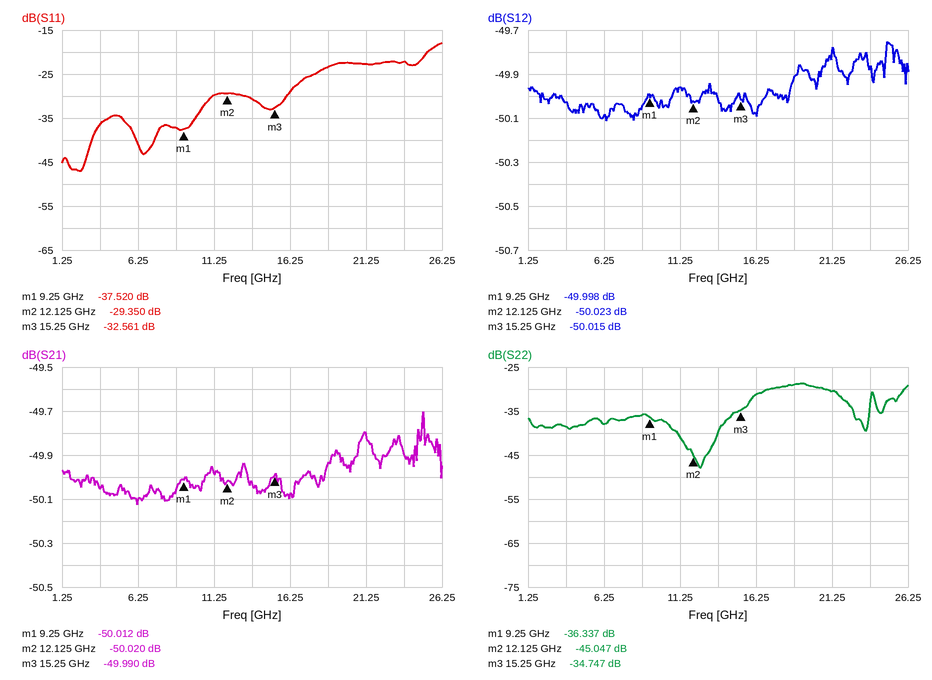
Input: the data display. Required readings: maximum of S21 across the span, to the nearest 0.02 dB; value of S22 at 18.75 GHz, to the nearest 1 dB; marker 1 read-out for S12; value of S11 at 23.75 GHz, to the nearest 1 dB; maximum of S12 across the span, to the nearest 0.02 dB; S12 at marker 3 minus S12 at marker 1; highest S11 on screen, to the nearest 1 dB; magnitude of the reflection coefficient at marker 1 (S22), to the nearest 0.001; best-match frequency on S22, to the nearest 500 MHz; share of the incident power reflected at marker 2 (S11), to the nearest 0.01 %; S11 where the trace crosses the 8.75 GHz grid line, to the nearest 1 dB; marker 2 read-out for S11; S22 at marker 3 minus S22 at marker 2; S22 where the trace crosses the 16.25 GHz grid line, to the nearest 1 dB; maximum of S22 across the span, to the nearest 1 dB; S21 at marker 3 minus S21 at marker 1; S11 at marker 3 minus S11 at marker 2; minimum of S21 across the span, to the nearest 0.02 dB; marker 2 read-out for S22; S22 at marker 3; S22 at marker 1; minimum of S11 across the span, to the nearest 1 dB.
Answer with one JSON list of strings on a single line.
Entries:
["-49.70 dB", "-29 dB", "-49.998 dB", "-22 dB", "-49.76 dB", "-0.017 dB", "-18 dB", "0.015", "12.5 GHz", "0.12 %", "-37 dB", "-29.350 dB", "10.300 dB", "-31 dB", "-29 dB", "0.022 dB", "-3.211 dB", "-50.12 dB", "-45.047 dB", "-34.747 dB", "-36.337 dB", "-47 dB"]
